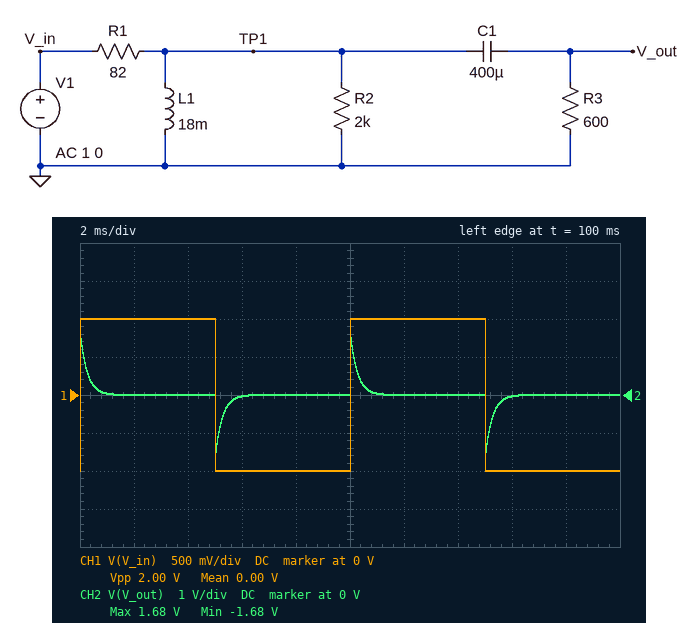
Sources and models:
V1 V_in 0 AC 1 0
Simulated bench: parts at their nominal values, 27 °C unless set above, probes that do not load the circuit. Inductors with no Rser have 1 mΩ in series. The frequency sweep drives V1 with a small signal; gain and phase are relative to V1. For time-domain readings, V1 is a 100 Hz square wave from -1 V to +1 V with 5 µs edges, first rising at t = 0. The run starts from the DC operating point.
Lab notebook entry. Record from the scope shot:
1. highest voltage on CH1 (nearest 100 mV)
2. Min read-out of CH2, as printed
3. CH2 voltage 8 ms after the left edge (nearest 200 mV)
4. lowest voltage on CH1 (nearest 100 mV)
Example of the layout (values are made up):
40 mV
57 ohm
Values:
1.0 V
-1.68 V
0 V
-1.0 V
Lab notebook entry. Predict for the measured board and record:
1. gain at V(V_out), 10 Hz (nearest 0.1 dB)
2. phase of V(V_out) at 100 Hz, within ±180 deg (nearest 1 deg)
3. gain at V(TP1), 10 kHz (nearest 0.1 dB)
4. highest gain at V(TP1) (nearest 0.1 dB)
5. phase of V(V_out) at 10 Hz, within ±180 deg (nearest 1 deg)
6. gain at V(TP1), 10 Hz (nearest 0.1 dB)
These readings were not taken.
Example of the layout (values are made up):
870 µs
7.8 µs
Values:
-37.2 dB
81 deg
-1.4 dB
-1.4 dB
93 deg
-37.2 dB
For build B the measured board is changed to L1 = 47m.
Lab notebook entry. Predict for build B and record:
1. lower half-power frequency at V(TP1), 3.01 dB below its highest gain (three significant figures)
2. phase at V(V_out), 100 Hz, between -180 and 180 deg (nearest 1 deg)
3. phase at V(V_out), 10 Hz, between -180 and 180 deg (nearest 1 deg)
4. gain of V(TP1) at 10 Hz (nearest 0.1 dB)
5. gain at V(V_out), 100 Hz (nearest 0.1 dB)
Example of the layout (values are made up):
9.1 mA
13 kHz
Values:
236 Hz
67 deg
91 deg
-28.9 dB
-9.6 dB
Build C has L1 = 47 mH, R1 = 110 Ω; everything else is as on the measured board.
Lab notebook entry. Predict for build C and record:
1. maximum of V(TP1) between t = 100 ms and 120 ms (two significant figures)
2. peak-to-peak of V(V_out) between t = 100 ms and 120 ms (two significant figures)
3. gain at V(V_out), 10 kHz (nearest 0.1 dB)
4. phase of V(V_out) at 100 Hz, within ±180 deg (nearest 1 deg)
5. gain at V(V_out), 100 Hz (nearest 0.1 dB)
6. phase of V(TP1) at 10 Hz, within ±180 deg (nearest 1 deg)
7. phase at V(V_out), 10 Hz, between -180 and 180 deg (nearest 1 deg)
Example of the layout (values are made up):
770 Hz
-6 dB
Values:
1.6 V
3.2 V
-1.9 dB
72 deg
-11.9 dB
88 deg
92 deg
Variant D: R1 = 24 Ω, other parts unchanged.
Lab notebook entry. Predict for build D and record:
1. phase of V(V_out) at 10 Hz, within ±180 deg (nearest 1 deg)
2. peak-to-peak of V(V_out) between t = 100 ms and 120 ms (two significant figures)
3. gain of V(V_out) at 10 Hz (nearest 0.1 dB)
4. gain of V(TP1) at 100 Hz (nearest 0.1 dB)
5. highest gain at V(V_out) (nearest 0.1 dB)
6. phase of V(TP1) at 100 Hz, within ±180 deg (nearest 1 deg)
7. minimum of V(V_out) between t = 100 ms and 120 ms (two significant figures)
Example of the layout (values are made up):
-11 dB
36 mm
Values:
91 deg
3.8 V
-26.6 dB
-7.5 dB
-0.4 dB
64 deg
-1.9 V
